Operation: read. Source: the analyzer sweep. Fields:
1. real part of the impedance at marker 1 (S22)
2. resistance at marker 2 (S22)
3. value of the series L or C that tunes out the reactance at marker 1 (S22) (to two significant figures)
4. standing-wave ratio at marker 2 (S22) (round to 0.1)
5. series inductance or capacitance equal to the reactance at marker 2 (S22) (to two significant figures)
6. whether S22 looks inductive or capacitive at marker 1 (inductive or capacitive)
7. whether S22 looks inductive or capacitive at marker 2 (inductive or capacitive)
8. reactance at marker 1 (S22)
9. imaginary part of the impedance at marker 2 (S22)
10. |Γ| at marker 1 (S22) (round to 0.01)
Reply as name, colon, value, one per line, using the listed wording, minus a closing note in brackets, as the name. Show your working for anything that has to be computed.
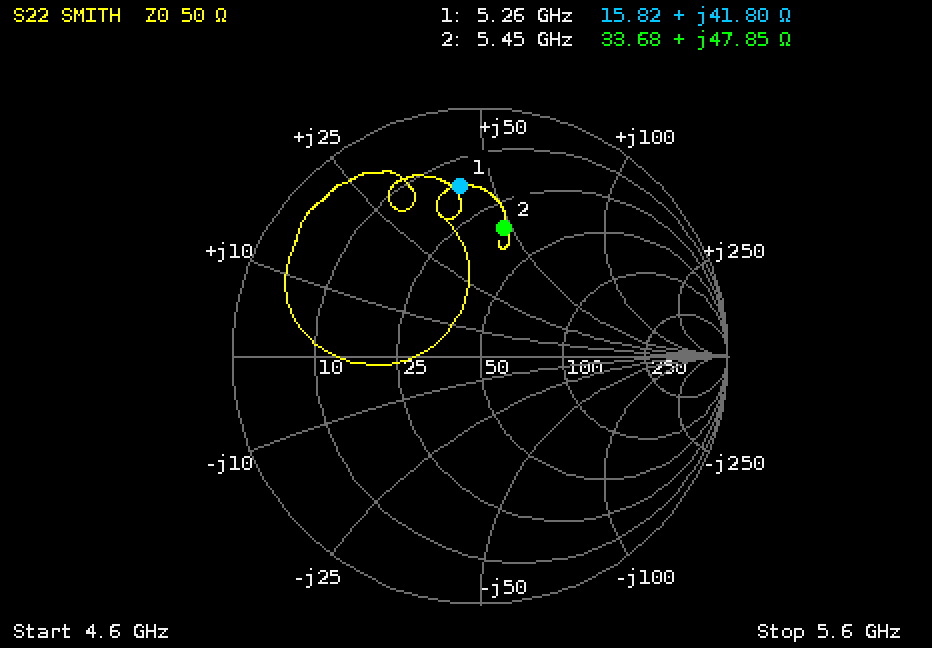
real part of the impedance at marker 1: 15.82 Ω
resistance at marker 2: 33.68 Ω
value of the series L or C that tunes out the reactance at marker 1 (S22): C = 1/(2π × 5.26 GHz × 41.8 Ω) ≈ 724 fF, so 720 fF to two significant figures
standing-wave ratio at marker 2 (S22): 3.2
series inductance or capacitance equal to the reactance at marker 2 (S22): L = 47.85 Ω/(2π × 5.45 GHz) ≈ 1.4 nH
whether S22 looks inductive or capacitive at marker 1: inductive
whether S22 looks inductive or capacitive at marker 2: inductive
reactance at marker 1: +41.80 Ω
imaginary part of the impedance at marker 2: +47.85 Ω
|Γ| at marker 1 (S22): 0.69
